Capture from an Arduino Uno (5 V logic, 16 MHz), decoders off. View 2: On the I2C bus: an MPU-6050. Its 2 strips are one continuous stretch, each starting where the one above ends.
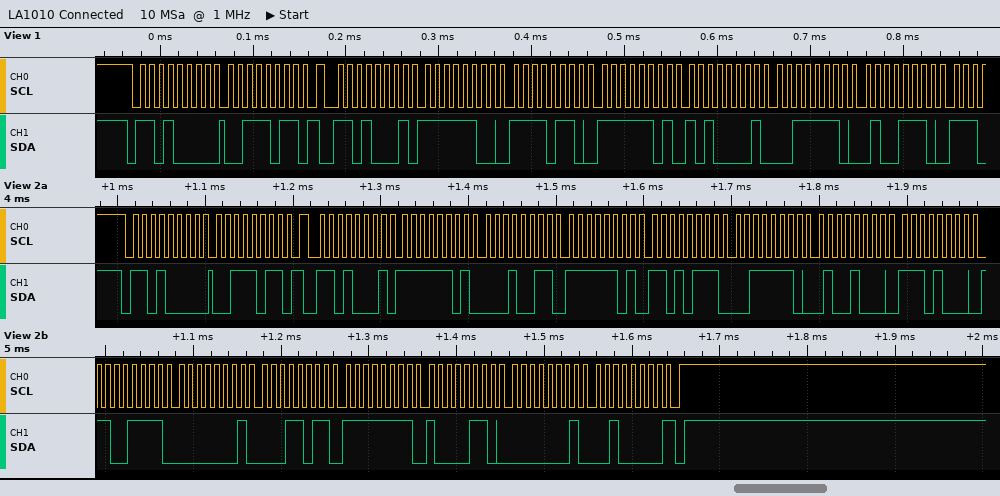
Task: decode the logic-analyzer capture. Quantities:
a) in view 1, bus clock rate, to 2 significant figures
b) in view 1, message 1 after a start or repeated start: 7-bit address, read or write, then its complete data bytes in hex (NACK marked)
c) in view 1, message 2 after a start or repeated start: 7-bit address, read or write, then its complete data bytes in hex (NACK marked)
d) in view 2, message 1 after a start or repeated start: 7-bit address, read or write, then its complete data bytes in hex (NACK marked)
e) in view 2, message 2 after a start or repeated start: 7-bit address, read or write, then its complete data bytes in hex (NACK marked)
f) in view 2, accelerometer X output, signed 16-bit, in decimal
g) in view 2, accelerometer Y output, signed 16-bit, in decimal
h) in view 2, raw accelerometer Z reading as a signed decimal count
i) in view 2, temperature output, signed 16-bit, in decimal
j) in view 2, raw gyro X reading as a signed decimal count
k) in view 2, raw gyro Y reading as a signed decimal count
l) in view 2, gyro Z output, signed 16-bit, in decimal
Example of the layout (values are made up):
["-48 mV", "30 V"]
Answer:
["100 kHz", "0x68 write: 3B", "0x68 read: FC F6 FD A1 3E 4E", "0x68 write: 3B", "0x68 read: FD 13 FD D7 3E 48 E8 CF 01 1B FF 86 01 20 NACK", "-749", "-553", "15944", "-5937", "283", "-122", "288"]
